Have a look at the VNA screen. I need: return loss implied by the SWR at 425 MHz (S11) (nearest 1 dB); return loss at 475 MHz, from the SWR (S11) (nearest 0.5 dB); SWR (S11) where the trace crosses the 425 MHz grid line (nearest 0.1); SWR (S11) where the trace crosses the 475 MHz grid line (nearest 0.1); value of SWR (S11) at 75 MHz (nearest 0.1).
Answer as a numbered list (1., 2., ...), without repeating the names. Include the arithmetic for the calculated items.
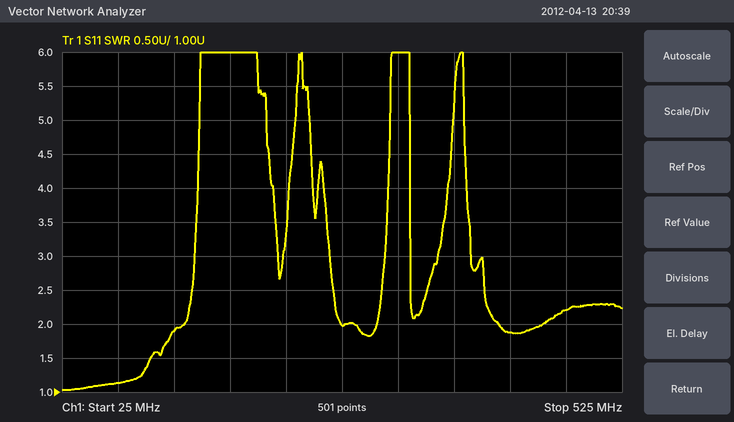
1. −20 log10((1.9 − 1)/(1.9 + 1)) ≈ 10 dB
2. −20 log10((2.2 − 1)/(2.2 + 1)) ≈ 8.5 dB
3. 1.9
4. 2.2
5. 1.1
